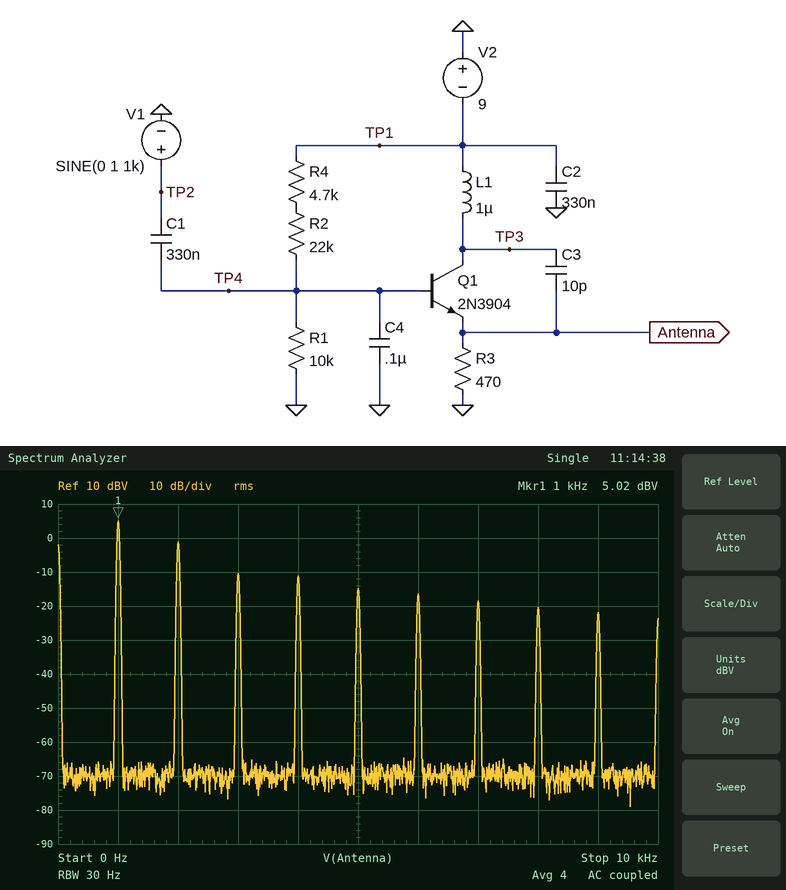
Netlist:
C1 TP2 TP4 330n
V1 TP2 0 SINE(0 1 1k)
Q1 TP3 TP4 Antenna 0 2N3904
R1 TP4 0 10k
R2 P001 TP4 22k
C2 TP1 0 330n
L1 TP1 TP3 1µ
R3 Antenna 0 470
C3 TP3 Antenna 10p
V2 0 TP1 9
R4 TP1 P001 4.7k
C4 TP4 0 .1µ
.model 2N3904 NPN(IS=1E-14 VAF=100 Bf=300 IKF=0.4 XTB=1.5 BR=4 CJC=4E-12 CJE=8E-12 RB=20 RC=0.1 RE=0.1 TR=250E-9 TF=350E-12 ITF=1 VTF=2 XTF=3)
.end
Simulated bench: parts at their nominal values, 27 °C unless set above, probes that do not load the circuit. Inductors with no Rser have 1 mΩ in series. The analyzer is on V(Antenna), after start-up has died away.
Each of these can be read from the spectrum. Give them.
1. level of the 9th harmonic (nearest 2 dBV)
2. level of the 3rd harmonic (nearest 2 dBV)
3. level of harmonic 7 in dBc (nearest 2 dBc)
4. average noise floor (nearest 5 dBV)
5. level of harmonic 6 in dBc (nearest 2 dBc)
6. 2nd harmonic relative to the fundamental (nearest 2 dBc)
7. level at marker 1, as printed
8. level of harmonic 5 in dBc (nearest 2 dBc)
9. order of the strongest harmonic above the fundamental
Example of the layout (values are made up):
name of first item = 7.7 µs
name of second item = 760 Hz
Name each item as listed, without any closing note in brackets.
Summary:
level of the 9th harmonic = -22 dBV
level of the 3rd harmonic = -10 dBV
level of harmonic 7 in dBc = -24 dBc
average noise floor = -70 dBV
level of harmonic 6 in dBc = -22 dBc
2nd harmonic relative to the fundamental = -6 dBc
level at marker 1, as printed = 5.02 dBV
level of harmonic 5 in dBc = -20 dBc
order of the strongest harmonic above the fundamental = 2
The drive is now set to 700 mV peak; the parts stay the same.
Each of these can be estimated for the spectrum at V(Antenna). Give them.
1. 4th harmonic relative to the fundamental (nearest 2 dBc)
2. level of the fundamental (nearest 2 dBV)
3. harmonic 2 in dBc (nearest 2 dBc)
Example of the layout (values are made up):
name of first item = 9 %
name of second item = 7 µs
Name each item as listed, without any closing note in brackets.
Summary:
4th harmonic relative to the fundamental = -20 dBc
level of the fundamental = 4 dBV
harmonic 2 in dBc = -10 dBc
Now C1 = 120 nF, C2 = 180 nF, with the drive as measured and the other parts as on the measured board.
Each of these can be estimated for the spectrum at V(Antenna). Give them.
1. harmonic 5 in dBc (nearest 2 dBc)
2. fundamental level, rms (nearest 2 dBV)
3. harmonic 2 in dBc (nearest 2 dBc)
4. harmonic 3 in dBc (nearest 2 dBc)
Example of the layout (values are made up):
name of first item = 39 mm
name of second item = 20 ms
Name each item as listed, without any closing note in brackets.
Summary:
harmonic 5 in dBc = -44 dBc
fundamental level, rms = 0 dBV
harmonic 2 in dBc = -28 dBc
harmonic 3 in dBc = -34 dBc
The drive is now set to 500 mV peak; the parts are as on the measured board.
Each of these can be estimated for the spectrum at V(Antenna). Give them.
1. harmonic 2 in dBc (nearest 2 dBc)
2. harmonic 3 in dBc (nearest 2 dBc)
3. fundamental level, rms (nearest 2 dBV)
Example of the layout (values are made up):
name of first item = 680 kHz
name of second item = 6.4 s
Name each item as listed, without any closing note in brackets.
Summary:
harmonic 2 in dBc = -16 dBc
harmonic 3 in dBc = -22 dBc
fundamental level, rms = 2 dBV
